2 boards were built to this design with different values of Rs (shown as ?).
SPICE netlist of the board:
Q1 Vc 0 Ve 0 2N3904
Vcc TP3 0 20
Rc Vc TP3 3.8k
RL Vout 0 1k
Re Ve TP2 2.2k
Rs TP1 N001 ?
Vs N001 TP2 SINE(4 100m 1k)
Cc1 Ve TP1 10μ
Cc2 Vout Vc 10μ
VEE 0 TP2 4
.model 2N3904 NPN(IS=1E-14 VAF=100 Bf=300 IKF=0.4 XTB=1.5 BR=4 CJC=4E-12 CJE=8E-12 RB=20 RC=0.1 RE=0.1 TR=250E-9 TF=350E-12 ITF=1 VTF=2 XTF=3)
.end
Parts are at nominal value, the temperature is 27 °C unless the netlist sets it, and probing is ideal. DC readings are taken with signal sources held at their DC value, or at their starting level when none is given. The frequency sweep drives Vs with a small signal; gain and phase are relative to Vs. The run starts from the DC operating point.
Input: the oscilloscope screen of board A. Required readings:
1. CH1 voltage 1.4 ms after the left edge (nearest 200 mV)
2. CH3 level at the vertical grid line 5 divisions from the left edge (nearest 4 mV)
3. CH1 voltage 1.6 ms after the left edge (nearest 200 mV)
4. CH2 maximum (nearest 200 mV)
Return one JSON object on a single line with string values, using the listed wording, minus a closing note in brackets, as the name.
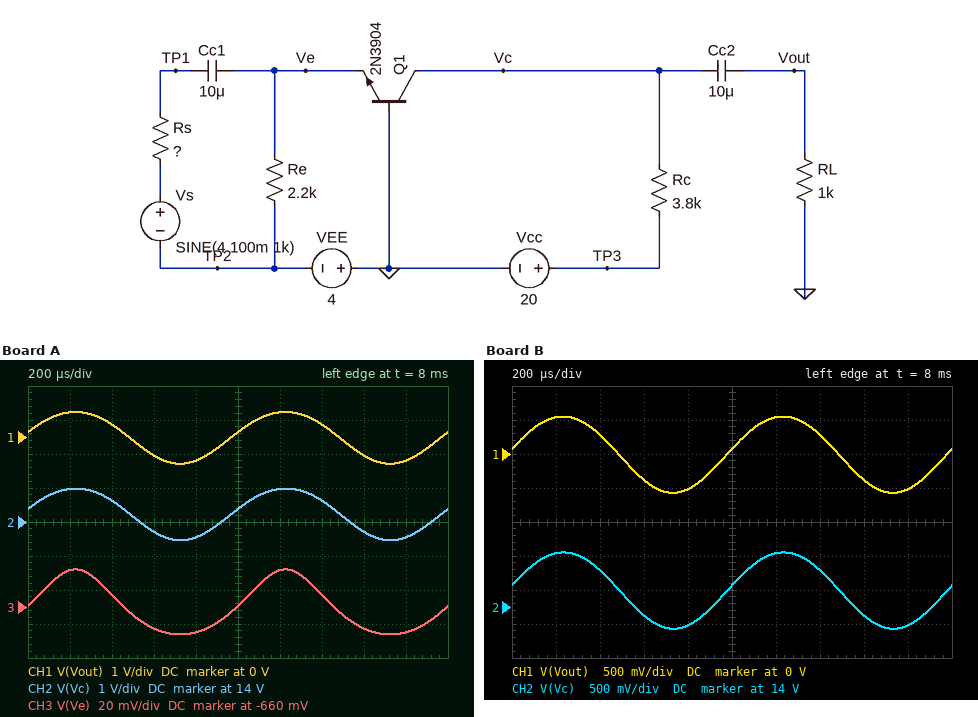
{"CH1 voltage 1.4 ms after the left edge": "400 mV", "CH3 level at the vertical grid line 5 divisions from the left edge": "-660 mV", "CH1 voltage 1.6 ms after the left edge": "-600 mV", "CH2 maximum": "15.0 V"}
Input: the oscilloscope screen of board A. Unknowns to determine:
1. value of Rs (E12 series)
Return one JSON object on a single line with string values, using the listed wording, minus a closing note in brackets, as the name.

{"value of Rs": "82 Ω"}
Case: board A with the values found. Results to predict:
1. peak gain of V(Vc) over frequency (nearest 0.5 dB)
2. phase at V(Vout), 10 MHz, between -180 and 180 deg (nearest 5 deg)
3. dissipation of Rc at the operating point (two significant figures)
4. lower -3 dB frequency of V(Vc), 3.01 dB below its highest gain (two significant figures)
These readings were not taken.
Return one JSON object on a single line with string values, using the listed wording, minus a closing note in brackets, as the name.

{"peak gain of V(Vc) over frequency": "18.0 dB", "phase at V(Vout), 10 MHz, between -180 and 180 deg": "-5 deg", "dissipation of Rc at the operating point": "8.7 mW", "lower -3 dB frequency of V(Vc), 3.01 dB below its highest gain": "160 Hz"}
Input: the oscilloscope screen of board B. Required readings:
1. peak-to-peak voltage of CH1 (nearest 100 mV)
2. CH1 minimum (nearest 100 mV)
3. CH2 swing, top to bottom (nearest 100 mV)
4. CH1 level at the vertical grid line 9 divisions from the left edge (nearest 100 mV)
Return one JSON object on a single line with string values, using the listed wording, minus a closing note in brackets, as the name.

{"peak-to-peak voltage of CH1": "1.1 V", "CH1 minimum": "-600 mV", "CH2 swing, top to bottom": "1.1 V", "CH1 level at the vertical grid line 9 divisions from the left edge": "-500 mV"}
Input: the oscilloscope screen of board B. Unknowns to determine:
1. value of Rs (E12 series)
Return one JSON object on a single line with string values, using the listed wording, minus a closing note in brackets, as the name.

{"value of Rs": "120 Ω"}
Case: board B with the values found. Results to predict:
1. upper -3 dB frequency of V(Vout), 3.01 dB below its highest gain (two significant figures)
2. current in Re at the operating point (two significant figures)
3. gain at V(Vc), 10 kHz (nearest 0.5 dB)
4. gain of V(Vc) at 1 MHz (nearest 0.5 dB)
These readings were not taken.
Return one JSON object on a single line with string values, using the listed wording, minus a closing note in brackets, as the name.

{"upper -3 dB frequency of V(Vout), 3.01 dB below its highest gain": "97 MHz", "current in Re at the operating point": "1.5 mA", "gain at V(Vc), 10 kHz": "15.0 dB", "gain of V(Vc) at 1 MHz": "15.0 dB"}
